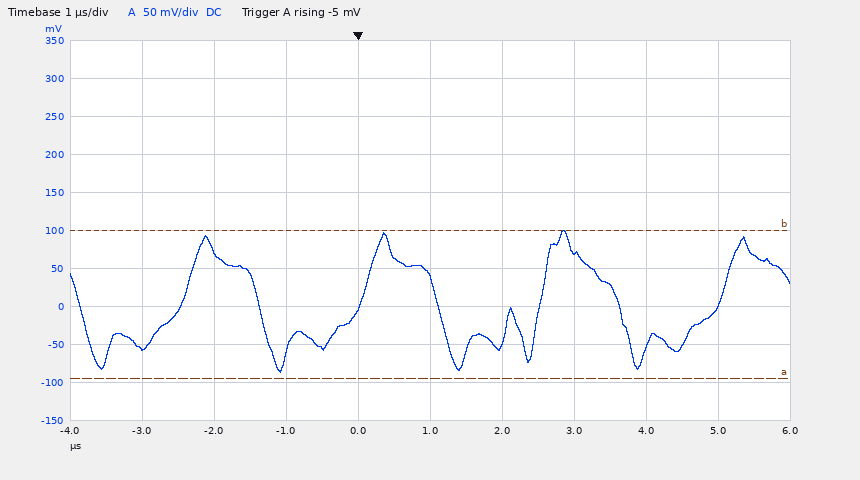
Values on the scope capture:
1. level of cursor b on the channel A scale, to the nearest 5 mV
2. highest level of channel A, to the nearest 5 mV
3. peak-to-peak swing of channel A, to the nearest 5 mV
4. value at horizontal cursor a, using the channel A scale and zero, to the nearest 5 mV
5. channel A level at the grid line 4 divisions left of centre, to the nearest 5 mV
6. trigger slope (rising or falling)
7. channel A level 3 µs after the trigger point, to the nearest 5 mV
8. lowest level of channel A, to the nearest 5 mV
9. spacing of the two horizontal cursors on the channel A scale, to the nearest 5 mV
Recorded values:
100 mV
100 mV
185 mV
-95 mV
-55 mV
rising
70 mV
-85 mV
195 mV
